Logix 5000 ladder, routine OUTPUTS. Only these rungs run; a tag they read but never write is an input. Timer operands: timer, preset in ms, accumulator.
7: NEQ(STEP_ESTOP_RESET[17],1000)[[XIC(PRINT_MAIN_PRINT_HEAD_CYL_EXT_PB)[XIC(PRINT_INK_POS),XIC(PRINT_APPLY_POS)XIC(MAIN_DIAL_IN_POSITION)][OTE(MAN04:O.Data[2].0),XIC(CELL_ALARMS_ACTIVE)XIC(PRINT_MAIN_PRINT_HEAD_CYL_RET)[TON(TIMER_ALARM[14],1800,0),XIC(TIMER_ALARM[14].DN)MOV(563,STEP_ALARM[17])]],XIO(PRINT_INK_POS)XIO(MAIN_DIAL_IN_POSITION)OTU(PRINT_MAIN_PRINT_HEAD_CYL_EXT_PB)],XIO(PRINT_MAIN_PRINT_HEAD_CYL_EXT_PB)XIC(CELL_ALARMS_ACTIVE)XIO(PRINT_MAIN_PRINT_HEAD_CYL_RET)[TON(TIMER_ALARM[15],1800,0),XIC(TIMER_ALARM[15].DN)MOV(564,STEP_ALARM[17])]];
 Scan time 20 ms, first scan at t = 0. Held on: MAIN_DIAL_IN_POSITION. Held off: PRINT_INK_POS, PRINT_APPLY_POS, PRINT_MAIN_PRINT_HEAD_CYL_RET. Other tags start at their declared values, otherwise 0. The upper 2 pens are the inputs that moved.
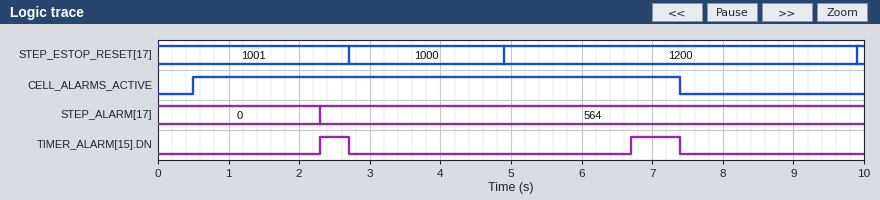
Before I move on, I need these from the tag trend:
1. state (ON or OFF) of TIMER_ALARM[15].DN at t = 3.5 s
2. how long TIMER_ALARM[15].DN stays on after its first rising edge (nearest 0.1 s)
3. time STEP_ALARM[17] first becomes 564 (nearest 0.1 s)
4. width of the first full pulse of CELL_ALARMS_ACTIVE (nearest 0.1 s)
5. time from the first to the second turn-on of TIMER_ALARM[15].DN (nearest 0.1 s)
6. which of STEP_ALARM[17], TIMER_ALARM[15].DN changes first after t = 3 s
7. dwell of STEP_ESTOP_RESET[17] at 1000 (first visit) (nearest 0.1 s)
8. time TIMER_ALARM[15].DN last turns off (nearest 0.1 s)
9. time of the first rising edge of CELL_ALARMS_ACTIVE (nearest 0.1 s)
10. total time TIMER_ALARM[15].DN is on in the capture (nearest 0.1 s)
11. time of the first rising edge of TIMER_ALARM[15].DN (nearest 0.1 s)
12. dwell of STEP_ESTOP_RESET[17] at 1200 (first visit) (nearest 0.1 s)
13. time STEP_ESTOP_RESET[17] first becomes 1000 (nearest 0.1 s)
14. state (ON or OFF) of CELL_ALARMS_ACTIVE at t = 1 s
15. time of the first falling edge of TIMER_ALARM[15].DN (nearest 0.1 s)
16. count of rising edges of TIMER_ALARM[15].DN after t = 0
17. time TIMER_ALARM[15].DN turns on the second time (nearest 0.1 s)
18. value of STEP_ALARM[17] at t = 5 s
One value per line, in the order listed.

OFF
0.4 s
2.3 s
6.9 s
4.4 s
TIMER_ALARM[15].DN
2.2 s
7.4 s
0.5 s
1.1 s
2.3 s
5.0 s
2.7 s
ON
2.7 s
2
6.7 s
564
